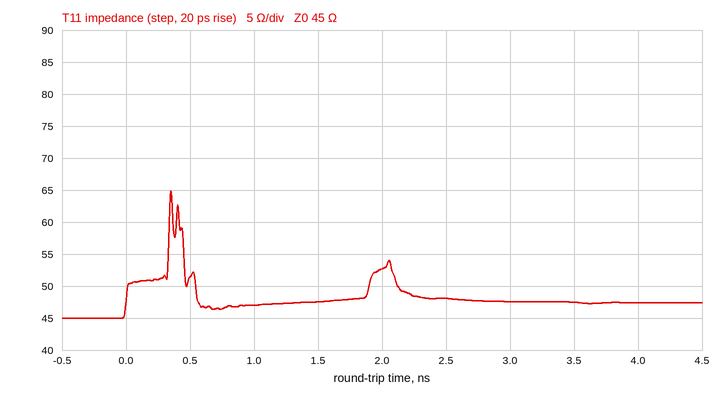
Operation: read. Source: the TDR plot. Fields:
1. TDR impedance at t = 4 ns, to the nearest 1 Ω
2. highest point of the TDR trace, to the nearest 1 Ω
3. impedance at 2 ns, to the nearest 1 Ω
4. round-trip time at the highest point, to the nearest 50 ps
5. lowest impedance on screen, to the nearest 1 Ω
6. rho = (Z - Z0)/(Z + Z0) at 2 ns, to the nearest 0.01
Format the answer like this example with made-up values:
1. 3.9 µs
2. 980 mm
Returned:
1. 47 Ω
2. 65 Ω
3. 53 Ω
4. 350 ps
5. 45 Ω
6. +0.08
